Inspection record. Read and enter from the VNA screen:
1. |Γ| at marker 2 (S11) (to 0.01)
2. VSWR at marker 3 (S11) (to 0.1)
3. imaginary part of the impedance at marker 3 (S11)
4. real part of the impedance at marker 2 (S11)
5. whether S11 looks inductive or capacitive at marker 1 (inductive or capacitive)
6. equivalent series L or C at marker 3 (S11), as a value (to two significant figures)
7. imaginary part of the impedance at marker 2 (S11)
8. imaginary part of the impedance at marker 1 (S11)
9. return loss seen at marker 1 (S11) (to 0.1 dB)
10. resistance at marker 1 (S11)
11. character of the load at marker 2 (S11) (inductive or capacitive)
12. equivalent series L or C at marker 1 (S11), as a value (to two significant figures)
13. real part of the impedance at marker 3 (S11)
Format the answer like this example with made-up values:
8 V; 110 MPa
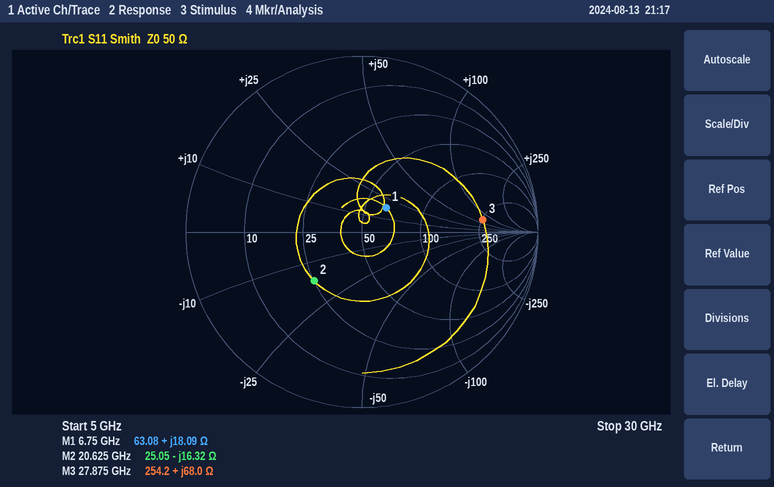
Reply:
0.39; 5.5; +68.0 Ω; 25.05 Ω; inductive; 390 pH; -16.32 Ω; +18.09 Ω; 14.2 dB; 63.08 Ω; capacitive; 430 pH; 254.2 Ω
